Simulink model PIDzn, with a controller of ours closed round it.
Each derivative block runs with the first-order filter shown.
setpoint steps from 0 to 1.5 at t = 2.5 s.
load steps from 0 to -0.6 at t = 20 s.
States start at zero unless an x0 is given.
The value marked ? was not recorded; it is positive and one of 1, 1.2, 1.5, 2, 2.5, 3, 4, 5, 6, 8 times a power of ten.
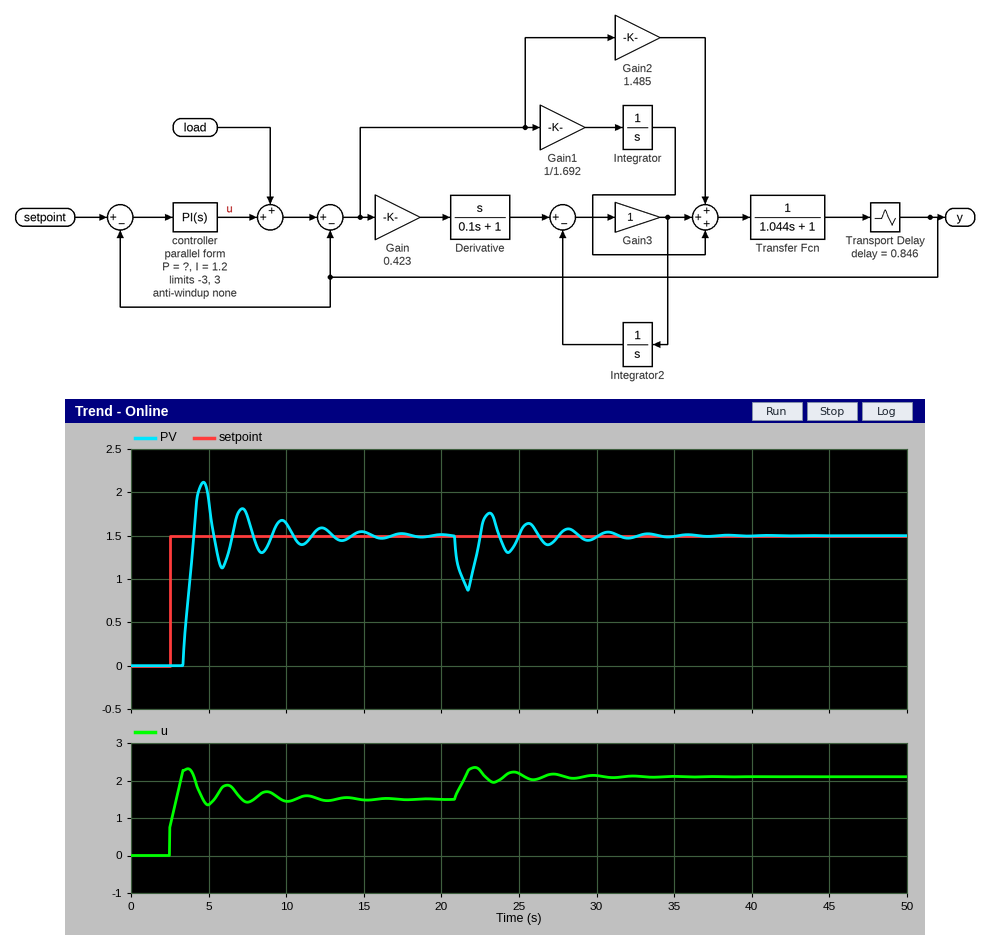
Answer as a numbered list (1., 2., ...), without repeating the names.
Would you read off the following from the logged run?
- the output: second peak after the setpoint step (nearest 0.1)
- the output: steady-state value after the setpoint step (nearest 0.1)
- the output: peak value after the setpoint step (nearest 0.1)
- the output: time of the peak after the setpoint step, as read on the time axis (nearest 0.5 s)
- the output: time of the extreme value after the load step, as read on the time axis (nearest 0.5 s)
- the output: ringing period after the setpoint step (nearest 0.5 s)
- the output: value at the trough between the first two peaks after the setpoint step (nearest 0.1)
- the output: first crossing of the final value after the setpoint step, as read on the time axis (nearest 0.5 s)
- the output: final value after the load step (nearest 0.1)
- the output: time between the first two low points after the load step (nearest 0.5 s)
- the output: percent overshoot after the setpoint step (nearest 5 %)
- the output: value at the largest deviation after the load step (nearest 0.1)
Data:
1. 1.8
2. 1.5
3. 2.1
4. 4.5 s
5. 21.5 s
6. 2.5 s
7. 1.1
8. 4.0 s
9. 1.5
10. 2.5 s
11. 40 %
12. 0.9
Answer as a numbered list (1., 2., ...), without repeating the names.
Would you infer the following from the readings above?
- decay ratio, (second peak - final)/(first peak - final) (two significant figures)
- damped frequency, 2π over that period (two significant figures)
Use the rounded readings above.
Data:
1. 0.50
2. 2.5 rad/s
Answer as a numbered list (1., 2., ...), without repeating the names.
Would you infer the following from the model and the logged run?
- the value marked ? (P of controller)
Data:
1. 0.5
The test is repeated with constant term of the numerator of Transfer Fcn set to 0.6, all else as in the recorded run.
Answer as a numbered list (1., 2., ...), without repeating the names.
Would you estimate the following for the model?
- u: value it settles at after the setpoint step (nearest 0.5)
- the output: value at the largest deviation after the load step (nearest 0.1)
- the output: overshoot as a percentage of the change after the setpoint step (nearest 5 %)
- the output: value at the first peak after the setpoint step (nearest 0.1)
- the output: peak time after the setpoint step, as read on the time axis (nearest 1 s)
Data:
1. 1.5
2. 1.1
3. 25 %
4. 1.9
5. 6 s
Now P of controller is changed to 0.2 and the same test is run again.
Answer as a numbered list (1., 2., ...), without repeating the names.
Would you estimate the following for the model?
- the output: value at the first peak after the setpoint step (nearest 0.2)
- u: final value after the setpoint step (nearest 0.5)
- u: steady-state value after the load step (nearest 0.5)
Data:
1. 2.2
2. 1.5
3. 2.0
